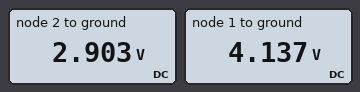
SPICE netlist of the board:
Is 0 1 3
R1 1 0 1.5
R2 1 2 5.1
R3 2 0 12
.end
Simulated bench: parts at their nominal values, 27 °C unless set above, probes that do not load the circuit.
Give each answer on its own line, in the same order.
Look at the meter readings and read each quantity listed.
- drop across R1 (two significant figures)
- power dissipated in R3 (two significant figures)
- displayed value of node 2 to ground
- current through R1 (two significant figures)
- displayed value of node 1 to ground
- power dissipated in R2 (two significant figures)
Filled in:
4.1 V
700 mW
2.903 V
2.8 A
4.137 V
300 mW
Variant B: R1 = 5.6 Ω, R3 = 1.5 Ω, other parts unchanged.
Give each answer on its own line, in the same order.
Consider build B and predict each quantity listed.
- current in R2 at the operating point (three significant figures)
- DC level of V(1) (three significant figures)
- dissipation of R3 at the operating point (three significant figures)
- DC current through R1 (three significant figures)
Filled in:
1.38 A
9.09 V
2.84 W
1.62 A
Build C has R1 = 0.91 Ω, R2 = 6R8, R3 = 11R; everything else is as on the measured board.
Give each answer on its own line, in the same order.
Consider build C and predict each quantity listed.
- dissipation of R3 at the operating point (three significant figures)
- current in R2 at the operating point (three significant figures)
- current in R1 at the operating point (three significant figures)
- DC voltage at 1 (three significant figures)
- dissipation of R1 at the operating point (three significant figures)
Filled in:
234 mW
146 mA
2.85 A
2.60 V
7.41 W
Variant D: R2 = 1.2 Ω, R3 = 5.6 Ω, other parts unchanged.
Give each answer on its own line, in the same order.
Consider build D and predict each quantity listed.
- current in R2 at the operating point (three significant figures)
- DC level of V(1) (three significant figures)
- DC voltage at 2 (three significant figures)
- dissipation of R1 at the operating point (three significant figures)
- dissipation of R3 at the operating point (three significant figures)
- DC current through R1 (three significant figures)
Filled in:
542 mA
3.69 V
3.04 V
9.06 W
1.65 W
2.46 A
